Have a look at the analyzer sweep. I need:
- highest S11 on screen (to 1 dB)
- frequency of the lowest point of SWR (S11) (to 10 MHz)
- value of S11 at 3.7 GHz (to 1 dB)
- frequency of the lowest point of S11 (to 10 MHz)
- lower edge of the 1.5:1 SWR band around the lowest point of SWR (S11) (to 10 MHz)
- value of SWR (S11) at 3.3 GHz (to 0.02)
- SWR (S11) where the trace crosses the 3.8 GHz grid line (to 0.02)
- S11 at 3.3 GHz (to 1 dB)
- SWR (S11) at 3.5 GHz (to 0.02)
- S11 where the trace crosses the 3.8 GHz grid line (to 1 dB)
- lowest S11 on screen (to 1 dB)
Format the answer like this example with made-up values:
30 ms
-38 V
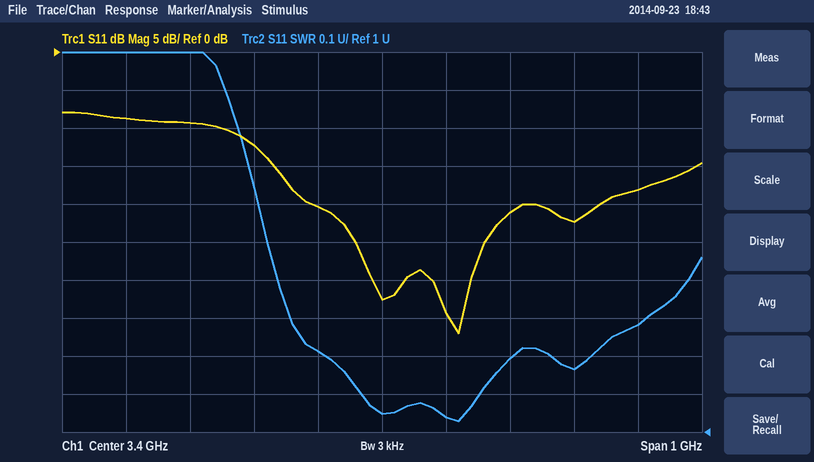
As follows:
-8 dB
3.52 GHz
-22 dB
3.52 GHz
3.22 GHz
1.22
1.28
-20 dB
1.04
-18 dB
-37 dB
